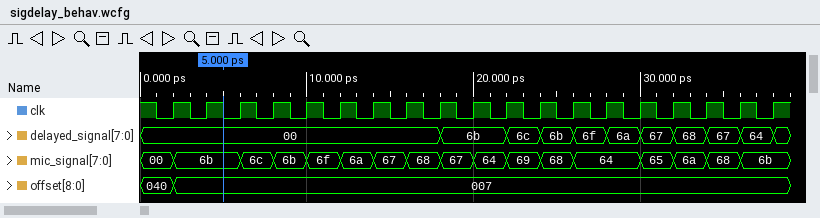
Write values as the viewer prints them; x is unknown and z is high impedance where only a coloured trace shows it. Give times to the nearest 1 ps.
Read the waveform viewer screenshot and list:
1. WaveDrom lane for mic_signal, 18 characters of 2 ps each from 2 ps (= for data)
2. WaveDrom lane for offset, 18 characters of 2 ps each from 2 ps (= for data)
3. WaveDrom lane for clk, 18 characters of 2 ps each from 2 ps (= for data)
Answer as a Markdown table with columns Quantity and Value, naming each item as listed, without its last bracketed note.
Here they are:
| Quantity | Value |
|---|---|
| WaveDrom lane for mic_signal, 18 characters of 2 ps each from 2 ps | {name: 'mic_signal', wave: '=.===========.====', data: '6b 6c 6b 6f 6a 67 68 67 64 69 68 64 65 6a 68 6b'} |
| WaveDrom lane for offset, 18 characters of 2 ps each from 2 ps | {name: 'offset', wave: '=.................', data: '007'} |
| WaveDrom lane for clk, 18 characters of 2 ps each from 2 ps | {name: 'clk', wave: 'p.................'} |
